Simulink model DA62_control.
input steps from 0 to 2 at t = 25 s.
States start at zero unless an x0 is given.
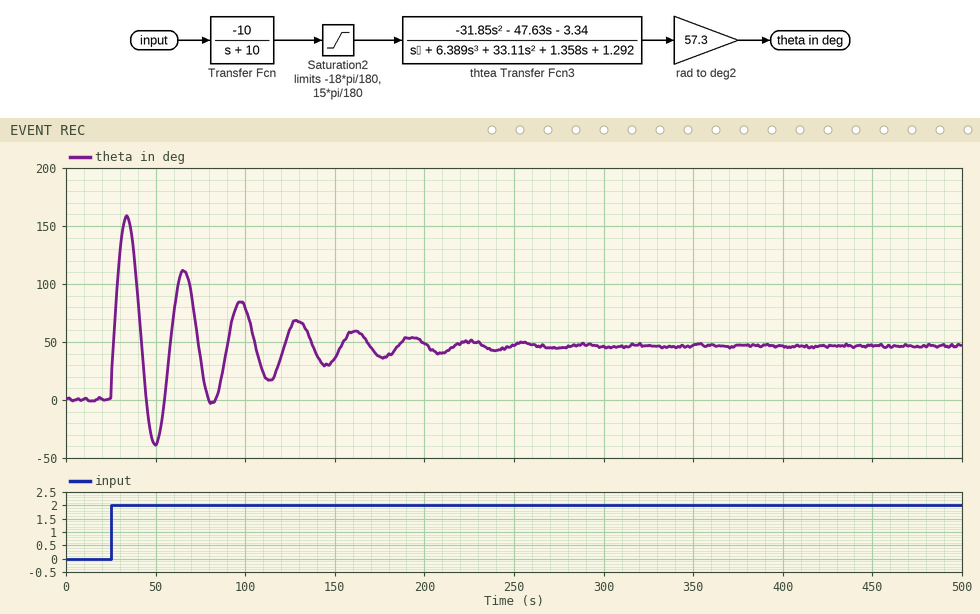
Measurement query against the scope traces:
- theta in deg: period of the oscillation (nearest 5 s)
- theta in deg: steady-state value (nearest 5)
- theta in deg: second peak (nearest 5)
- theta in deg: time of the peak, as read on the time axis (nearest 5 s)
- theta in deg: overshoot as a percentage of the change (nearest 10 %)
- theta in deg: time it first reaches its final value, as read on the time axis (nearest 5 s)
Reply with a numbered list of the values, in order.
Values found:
1. 30 s
2. 45
3. 110
4. 35 s
5. 240 %
6. 25 s
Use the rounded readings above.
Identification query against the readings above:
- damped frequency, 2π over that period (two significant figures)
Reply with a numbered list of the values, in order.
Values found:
1. 0.21 rad/s
